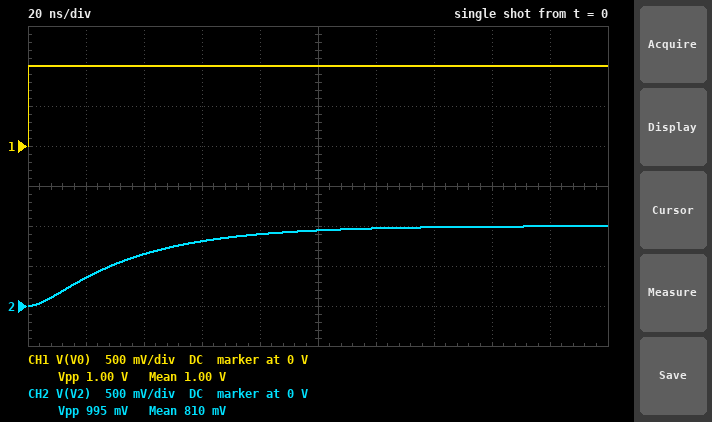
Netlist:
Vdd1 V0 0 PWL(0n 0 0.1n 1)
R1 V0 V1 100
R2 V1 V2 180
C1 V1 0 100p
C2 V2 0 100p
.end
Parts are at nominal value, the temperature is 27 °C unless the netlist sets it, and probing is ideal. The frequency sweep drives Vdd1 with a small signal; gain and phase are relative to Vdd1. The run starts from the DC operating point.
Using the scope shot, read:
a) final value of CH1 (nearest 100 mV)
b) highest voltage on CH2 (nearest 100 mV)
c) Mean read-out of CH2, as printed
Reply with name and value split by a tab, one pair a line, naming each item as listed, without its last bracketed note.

final value of CH1	1.0 V
highest voltage on CH2	1.0 V
Mean read-out of CH2, as printed	810 mV
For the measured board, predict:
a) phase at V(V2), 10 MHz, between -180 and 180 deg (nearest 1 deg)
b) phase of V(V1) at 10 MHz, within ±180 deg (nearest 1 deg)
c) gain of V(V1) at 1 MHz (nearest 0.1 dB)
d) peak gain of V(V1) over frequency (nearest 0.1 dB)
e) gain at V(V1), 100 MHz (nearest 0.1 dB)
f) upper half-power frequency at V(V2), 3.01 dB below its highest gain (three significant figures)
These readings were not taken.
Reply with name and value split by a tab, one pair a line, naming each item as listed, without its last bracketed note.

phase at V(V2), 10 MHz, between -180 and 180 deg	-83 deg
phase of V(V1) at 10 MHz, within ±180 deg	-35 deg
gain of V(V1) at 1 MHz	-0.1 dB
peak gain of V(V1) over frequency	0 dB
gain at V(V1), 100 MHz	-16.3 dB
upper half-power frequency at V(V2), 3.01 dB below its highest gain	4.77 MHz
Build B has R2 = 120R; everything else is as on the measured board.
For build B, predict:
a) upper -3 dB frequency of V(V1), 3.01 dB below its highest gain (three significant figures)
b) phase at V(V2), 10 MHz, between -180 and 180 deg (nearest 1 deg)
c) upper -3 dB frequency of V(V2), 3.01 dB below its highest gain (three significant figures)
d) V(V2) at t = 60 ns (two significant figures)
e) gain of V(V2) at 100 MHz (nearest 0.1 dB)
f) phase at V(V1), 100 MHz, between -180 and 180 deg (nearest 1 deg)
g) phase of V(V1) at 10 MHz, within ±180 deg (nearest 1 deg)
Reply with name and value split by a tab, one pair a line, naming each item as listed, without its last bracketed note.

upper -3 dB frequency of V(V1), 3.01 dB below its highest gain	6.96 MHz
phase at V(V2), 10 MHz, between -180 and 180 deg	-75 deg
upper -3 dB frequency of V(V2), 3.01 dB below its highest gain	5.62 MHz
V(V2) at t = 60 ns	860 mV
gain of V(V2) at 100 MHz	-34.1 dB
phase at V(V1), 100 MHz, between -180 and 180 deg	-74 deg
phase of V(V1) at 10 MHz, within ±180 deg	-38 deg
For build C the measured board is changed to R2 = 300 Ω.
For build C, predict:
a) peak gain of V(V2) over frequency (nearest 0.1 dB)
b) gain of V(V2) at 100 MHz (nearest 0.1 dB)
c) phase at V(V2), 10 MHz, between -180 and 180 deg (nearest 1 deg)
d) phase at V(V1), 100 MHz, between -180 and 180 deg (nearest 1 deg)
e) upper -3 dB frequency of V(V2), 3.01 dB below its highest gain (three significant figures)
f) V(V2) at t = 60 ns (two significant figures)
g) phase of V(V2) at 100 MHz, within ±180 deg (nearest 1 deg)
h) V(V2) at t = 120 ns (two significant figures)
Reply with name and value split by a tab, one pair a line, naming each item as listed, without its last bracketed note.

peak gain of V(V2) over frequency	0 dB
gain of V(V2) at 100 MHz	-41.7 dB
phase at V(V2), 10 MHz, between -180 and 180 deg	-93 deg
phase at V(V1), 100 MHz, between -180 and 180 deg	-78 deg
upper -3 dB frequency of V(V2), 3.01 dB below its highest gain	3.61 MHz
V(V2) at t = 60 ns	700 mV
phase of V(V2) at 100 MHz, within ±180 deg	-165 deg
V(V2) at t = 120 ns	930 mV
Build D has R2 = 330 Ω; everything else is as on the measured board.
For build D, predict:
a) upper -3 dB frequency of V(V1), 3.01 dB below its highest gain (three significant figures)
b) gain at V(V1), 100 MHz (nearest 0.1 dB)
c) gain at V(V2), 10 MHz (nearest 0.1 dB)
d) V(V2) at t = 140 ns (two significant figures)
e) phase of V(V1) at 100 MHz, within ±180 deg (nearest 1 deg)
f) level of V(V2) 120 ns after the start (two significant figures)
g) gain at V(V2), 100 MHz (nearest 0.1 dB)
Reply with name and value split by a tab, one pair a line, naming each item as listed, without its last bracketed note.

upper -3 dB frequency of V(V1), 3.01 dB below its highest gain	8.96 MHz
gain at V(V1), 100 MHz	-16.2 dB
gain at V(V2), 10 MHz	-10.5 dB
V(V2) at t = 140 ns	940 mV
phase of V(V1) at 100 MHz, within ±180 deg	-78 deg
level of V(V2) 120 ns after the start	910 mV
gain at V(V2), 100 MHz	-42.5 dB
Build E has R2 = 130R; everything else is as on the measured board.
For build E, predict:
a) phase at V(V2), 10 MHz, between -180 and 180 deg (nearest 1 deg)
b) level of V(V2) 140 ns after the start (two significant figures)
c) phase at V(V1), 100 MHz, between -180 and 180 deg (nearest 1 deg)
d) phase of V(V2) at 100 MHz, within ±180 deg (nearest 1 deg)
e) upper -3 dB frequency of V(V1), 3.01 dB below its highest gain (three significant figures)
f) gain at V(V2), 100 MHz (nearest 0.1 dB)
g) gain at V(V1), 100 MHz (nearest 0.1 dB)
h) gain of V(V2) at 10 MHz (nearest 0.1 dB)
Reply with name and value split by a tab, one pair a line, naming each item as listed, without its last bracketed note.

phase at V(V2), 10 MHz, between -180 and 180 deg	-77 deg
level of V(V2) 140 ns after the start	990 mV
phase at V(V1), 100 MHz, between -180 and 180 deg	-75 deg
phase of V(V2) at 100 MHz, within ±180 deg	-158 deg
upper -3 dB frequency of V(V1), 3.01 dB below its highest gain	6.96 MHz
gain at V(V2), 100 MHz	-34.7 dB
gain at V(V1), 100 MHz	-16.4 dB
gain of V(V2) at 10 MHz	-6.6 dB
